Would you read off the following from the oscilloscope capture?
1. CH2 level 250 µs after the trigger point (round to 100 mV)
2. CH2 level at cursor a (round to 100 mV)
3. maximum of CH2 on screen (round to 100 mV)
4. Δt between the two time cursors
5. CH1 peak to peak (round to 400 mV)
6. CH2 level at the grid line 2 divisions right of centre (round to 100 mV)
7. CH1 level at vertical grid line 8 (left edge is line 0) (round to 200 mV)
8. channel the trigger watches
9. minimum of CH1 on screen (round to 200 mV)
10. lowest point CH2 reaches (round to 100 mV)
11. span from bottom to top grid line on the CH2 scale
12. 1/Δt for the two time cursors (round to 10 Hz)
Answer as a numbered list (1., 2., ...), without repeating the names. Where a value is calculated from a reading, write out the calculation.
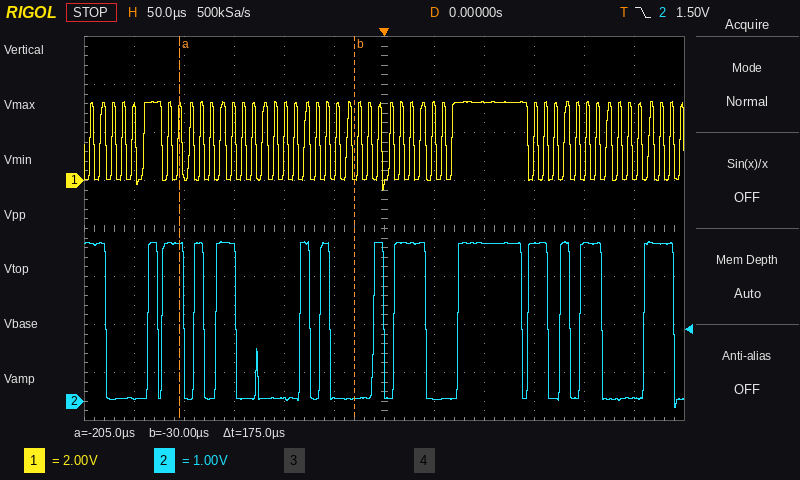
1. 100 mV
2. 3.2 V
3. 3.3 V
4. 175 µs
5. 3.6 V
6. 3.3 V
7. 3.2 V
8. CH2
9. -400 mV
10. -100 mV
11. 8 V
12. 1 / 175 µs ≈ 5.71 kHz
